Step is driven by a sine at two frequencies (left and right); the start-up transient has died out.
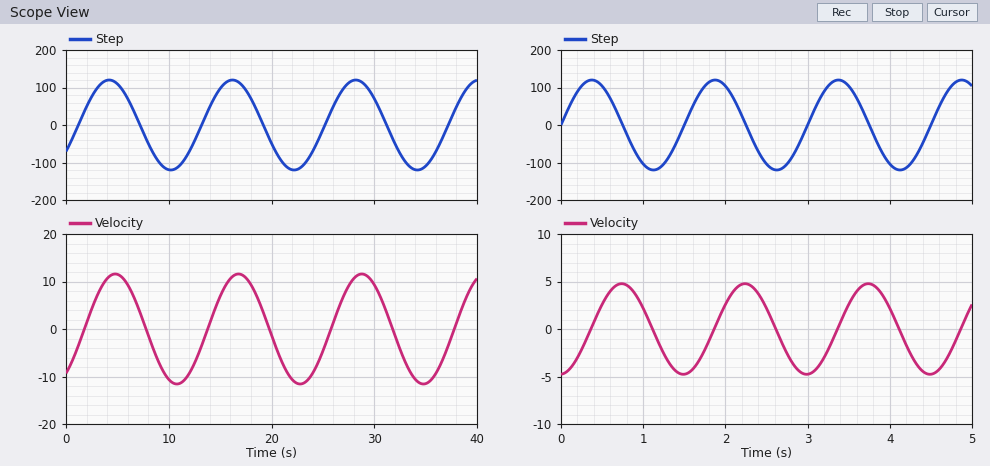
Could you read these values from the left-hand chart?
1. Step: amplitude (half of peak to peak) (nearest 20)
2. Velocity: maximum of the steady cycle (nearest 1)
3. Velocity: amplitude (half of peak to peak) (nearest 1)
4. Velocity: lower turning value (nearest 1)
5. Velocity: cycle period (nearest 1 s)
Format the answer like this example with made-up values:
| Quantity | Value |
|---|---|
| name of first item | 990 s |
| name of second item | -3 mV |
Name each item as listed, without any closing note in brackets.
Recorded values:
| Quantity | Value |
|---|---|
| Step: amplitude (half of peak to peak) | 120 |
| Velocity: maximum of the steady cycle | 12 |
| Velocity: amplitude (half of peak to peak) | 12 |
| Velocity: lower turning value | -12 |
| Velocity: cycle period | 12 s |
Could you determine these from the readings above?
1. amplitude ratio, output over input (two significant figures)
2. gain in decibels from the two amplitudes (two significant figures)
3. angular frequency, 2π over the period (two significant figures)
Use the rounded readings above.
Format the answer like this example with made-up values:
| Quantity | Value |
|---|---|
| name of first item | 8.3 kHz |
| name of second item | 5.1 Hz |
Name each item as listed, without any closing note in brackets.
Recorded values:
| Quantity | Value |
|---|---|
| amplitude ratio, output over input | 0.10 |
| gain in decibels from the two amplitudes | -20 dB |
| angular frequency, 2π over the period | 0.52 rad/s |
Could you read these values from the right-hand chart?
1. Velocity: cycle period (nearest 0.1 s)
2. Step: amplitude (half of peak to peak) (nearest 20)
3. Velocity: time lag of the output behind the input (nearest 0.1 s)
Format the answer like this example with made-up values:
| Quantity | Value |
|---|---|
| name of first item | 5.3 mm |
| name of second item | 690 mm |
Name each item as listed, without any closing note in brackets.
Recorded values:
| Quantity | Value |
|---|---|
| Velocity: cycle period | 1.5 s |
| Step: amplitude (half of peak to peak) | 120 |
| Velocity: time lag of the output behind the input | 0.4 s |
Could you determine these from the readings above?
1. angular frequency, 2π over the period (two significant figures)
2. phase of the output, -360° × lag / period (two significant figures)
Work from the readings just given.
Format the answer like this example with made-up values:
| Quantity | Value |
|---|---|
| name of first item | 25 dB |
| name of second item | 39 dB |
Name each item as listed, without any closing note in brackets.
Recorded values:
| Quantity | Value |
|---|---|
| angular frequency, 2π over the period | 4.2 rad/s |
| phase of the output, -360° × lag / period | -96° |
